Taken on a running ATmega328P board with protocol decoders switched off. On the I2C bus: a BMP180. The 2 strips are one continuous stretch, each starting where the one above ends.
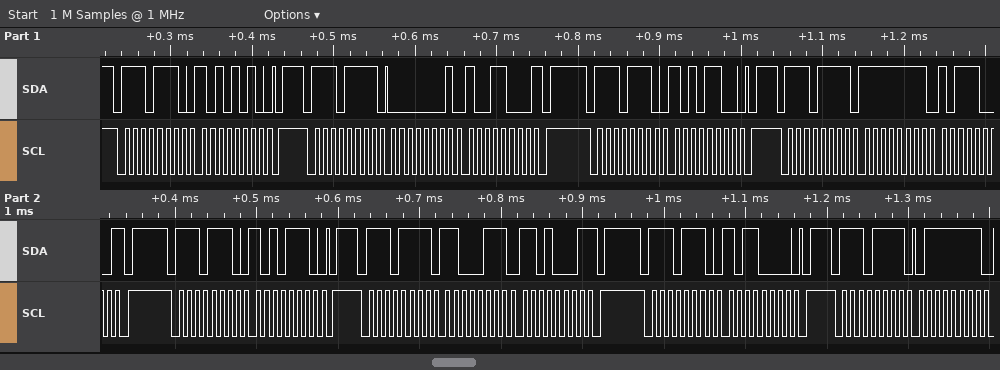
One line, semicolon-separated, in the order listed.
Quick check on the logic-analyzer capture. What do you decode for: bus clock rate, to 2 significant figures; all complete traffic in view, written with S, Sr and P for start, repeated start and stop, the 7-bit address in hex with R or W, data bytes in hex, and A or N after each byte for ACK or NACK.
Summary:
100 kHz; S 77W A AA A P S 77R A 01 A 98 N P S 77W A AC A P S 77R A FF A B8 N P S 77W A AE A P S 77R A C7 A D1 N P S 77W A B0 A P S 77R A 7F A
